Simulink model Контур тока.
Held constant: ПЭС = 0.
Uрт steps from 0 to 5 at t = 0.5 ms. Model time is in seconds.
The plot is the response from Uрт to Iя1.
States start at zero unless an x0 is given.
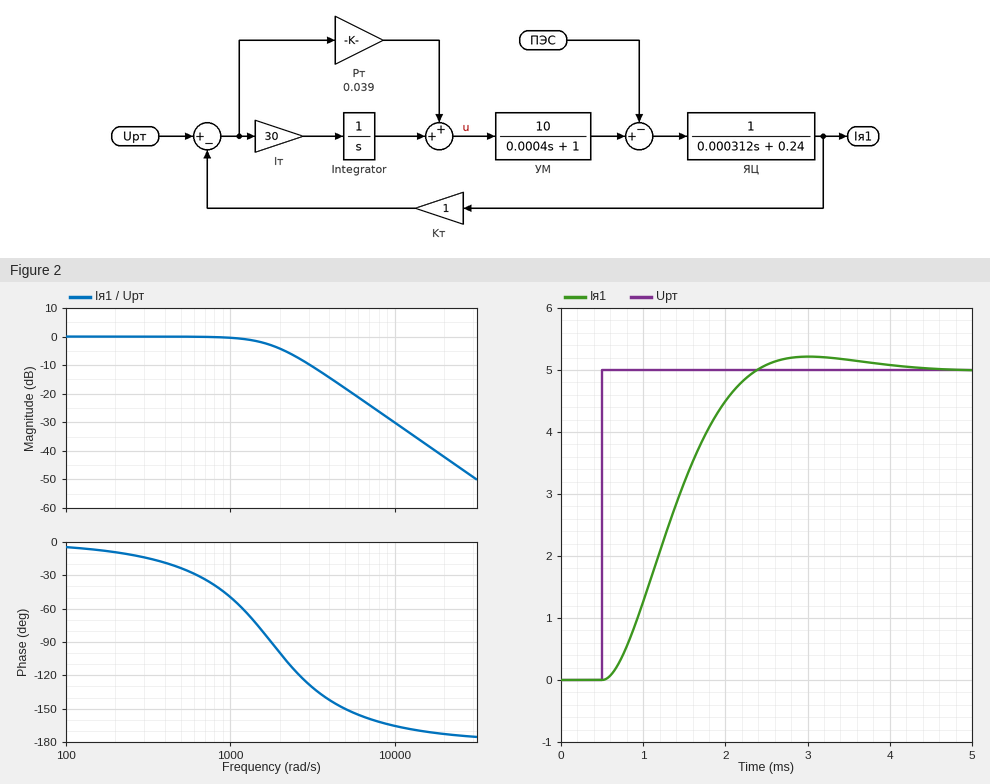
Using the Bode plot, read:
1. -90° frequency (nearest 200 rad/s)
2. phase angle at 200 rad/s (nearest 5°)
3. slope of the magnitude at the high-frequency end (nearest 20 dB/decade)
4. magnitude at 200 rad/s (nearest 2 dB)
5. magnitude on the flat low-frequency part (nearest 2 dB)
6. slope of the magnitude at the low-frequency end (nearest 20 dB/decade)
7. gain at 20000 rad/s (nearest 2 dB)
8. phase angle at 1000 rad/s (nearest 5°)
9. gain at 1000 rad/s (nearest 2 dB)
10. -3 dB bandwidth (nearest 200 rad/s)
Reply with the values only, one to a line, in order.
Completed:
1800 rad/s
-10°
-40 dB/decade
0 dB
0 dB
0 dB/decade
-42 dB
-50°
0 dB
1800 rad/s
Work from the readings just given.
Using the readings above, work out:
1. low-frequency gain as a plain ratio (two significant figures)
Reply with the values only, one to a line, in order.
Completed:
1.0
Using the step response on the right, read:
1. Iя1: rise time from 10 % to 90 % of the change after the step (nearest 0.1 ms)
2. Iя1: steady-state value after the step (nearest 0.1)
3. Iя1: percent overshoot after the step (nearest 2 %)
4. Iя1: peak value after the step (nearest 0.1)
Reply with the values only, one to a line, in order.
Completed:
1.2 ms
5.0
4 %
5.2
